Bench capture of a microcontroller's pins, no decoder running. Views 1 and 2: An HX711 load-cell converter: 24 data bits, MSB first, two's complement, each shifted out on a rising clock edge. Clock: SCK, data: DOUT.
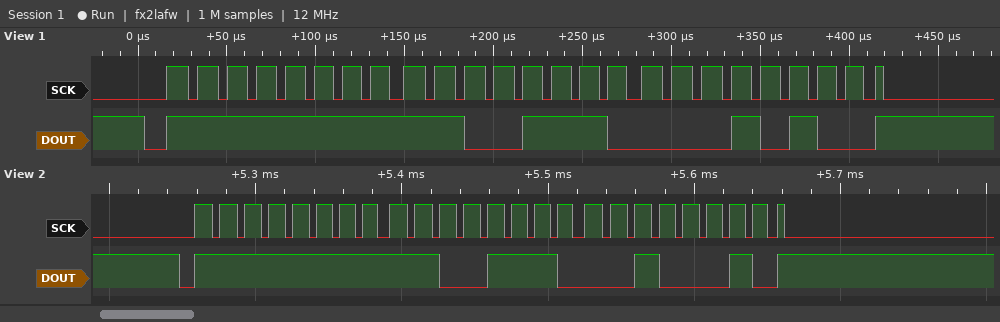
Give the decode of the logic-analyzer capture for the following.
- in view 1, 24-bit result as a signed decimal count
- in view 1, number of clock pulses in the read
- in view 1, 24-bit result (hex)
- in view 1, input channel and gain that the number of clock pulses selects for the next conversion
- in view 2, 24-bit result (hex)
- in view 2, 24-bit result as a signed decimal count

-12780
25
0xFFCE14
channel A, gain 128
0xFFCE22
-12766
